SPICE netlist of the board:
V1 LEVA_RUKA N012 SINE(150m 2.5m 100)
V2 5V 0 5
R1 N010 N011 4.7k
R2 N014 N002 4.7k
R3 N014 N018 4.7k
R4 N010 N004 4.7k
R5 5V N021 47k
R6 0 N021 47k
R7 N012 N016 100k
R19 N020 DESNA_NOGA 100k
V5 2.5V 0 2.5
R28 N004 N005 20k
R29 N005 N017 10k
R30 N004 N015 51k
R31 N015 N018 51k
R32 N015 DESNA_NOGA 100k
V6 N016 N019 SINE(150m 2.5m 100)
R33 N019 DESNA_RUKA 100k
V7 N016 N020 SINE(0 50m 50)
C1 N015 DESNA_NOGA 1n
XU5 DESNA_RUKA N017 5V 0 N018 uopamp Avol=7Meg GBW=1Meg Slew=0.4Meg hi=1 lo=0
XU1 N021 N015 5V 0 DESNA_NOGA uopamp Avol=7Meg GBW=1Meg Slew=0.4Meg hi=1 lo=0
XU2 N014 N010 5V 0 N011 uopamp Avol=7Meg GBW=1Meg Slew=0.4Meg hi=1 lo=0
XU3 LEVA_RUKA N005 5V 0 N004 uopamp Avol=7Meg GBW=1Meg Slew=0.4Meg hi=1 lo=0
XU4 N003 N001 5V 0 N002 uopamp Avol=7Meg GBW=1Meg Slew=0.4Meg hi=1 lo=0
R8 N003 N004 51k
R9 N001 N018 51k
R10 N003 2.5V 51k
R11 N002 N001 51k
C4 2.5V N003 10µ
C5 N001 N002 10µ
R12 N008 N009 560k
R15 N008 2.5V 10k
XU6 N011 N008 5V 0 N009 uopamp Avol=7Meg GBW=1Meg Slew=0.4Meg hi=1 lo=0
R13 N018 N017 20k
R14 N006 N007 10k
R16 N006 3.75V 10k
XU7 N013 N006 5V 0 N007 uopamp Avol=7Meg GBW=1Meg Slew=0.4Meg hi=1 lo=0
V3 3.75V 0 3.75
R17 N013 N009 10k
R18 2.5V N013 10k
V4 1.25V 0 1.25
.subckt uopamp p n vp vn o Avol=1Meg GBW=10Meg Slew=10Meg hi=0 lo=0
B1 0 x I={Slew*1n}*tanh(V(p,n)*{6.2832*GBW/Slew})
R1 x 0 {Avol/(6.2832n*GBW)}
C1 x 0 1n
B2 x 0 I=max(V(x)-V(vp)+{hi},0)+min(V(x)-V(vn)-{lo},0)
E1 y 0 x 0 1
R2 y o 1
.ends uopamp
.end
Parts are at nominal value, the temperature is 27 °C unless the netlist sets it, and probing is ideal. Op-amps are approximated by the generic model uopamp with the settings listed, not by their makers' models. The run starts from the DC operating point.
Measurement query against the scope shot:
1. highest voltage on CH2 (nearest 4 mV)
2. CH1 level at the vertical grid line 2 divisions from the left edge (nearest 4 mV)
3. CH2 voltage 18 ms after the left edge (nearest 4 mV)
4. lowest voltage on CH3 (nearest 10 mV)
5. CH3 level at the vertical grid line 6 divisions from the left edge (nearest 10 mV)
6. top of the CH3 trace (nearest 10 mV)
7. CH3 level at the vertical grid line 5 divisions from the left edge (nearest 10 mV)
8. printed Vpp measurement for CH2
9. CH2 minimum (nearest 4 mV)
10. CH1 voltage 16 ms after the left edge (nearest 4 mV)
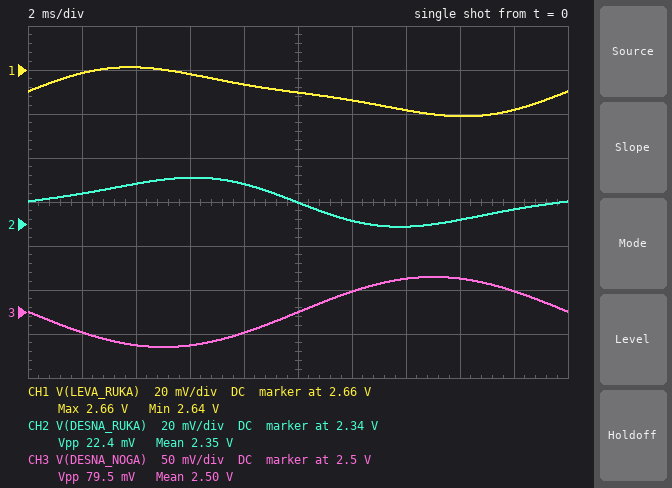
2.360 V
2.660 V
2.348 V
2.46 V
2.52 V
2.54 V
2.50 V
22.4 mV
2.340 V
2.640 V
